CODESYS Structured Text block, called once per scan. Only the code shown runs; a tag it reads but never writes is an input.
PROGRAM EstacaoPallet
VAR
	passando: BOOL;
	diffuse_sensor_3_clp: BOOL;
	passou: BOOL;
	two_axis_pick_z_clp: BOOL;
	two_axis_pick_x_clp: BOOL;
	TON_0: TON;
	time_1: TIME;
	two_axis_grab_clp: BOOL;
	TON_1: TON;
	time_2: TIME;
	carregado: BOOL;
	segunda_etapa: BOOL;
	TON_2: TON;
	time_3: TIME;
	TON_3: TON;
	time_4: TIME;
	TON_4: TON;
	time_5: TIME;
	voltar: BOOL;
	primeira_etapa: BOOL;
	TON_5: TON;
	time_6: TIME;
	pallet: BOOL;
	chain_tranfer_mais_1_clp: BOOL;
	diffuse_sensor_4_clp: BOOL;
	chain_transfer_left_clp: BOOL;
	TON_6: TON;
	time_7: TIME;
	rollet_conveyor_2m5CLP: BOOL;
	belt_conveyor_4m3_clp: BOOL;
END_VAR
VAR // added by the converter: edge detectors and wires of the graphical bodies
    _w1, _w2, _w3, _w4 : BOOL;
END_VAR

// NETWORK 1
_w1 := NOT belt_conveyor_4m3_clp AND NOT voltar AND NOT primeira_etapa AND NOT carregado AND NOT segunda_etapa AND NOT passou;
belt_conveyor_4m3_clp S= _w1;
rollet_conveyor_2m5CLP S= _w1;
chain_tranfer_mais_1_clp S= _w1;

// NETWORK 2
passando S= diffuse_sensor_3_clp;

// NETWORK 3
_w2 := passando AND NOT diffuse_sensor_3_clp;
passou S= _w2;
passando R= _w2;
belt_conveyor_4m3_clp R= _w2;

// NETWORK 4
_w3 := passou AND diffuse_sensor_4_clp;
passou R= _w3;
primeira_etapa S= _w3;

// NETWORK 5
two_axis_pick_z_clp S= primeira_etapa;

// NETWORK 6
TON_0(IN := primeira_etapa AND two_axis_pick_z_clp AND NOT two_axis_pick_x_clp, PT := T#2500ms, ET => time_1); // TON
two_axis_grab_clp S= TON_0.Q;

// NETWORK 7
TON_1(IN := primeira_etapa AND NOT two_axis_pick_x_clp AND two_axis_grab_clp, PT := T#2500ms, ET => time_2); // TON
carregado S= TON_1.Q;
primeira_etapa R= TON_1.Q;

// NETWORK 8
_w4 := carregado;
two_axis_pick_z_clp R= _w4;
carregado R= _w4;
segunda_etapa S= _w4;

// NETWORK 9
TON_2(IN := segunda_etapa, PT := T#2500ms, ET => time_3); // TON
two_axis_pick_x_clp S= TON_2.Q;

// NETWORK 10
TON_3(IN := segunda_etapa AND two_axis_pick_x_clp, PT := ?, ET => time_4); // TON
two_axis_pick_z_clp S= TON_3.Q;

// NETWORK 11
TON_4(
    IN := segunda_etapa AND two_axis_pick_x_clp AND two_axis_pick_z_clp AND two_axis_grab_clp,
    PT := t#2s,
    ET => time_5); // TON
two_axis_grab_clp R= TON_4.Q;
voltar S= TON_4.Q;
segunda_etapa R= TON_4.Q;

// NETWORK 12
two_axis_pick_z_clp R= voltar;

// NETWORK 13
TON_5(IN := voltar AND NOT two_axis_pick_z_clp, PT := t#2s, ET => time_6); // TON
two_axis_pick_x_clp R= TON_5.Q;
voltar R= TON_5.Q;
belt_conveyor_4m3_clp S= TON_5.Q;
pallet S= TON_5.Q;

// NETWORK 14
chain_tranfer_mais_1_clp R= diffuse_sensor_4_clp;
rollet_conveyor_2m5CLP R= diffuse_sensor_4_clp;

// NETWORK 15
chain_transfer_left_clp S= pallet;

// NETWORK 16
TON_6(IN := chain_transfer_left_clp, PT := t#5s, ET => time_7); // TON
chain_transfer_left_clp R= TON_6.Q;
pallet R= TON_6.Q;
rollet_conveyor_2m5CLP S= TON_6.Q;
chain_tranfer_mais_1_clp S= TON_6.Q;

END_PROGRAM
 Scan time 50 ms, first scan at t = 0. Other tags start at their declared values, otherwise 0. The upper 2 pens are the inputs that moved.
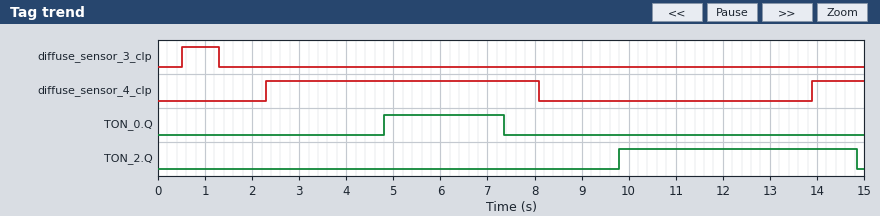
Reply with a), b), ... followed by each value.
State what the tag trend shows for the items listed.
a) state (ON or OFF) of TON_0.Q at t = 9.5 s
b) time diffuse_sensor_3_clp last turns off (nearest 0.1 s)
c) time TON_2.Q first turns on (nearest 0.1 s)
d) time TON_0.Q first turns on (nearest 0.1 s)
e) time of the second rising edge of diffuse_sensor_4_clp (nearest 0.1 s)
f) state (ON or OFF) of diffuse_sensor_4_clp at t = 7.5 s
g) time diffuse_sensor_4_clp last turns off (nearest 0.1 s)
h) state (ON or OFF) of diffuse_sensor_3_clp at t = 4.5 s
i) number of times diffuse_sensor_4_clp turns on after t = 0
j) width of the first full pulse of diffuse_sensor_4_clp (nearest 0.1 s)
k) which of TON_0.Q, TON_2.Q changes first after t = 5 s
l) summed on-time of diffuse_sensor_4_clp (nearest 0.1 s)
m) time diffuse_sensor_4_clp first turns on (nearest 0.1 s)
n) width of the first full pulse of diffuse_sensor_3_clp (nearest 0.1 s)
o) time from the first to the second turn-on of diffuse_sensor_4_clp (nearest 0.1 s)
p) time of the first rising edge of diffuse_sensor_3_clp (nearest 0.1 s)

a) OFF
b) 1.3 s
c) 9.8 s
d) 4.8 s
e) 13.9 s
f) ON
g) 8.1 s
h) OFF
i) 2
j) 5.8 s
k) TON_0.Q
l) 6.9 s
m) 2.3 s
n) 0.8 s
o) 11.6 s
p) 0.5 s
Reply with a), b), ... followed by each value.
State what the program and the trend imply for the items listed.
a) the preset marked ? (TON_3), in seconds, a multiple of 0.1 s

a) 3.0 s
